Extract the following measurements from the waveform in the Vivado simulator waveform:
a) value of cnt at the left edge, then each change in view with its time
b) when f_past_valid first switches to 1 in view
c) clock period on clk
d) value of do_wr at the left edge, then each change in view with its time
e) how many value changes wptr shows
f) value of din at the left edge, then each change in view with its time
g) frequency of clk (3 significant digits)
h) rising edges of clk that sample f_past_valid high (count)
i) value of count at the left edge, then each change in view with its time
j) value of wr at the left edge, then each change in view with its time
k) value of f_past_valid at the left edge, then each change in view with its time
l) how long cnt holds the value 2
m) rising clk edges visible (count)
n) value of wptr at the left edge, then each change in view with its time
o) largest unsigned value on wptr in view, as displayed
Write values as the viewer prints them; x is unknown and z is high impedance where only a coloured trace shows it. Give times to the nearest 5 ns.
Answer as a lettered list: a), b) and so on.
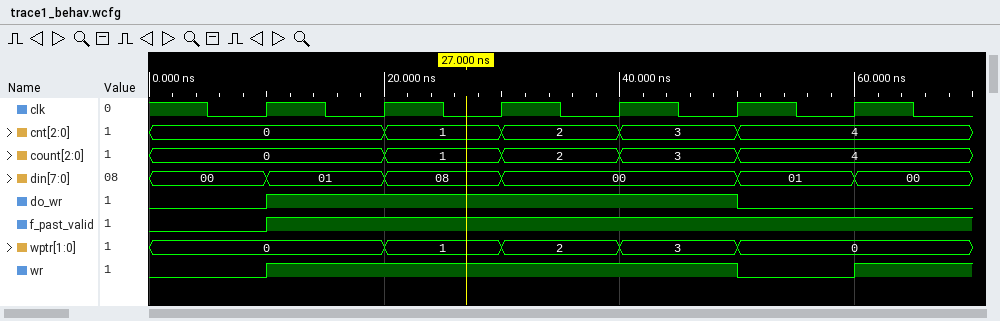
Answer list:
a) 0, 1 at 20 ns, 2 at 30 ns, 3 at 40 ns, 4 at 50 ns
b) 10 ns
c) 10 ns
d) 0, 1 at 10 ns, 0 at 50 ns
e) 4
f) 00, 01 at 10 ns, 08 at 20 ns, 00 at 30 ns, 01 at 50 ns, 00 at 60 ns
g) 100 MHz
h) 5
i) 0, 1 at 20 ns, 2 at 30 ns, 3 at 40 ns, 4 at 50 ns
j) 0, 1 at 10 ns, 0 at 50 ns, 1 at 60 ns
k) 0, 1 at 10 ns
l) 10 ns
m) 6
n) 0, 1 at 20 ns, 2 at 30 ns, 3 at 40 ns, 0 at 50 ns
o) 3
